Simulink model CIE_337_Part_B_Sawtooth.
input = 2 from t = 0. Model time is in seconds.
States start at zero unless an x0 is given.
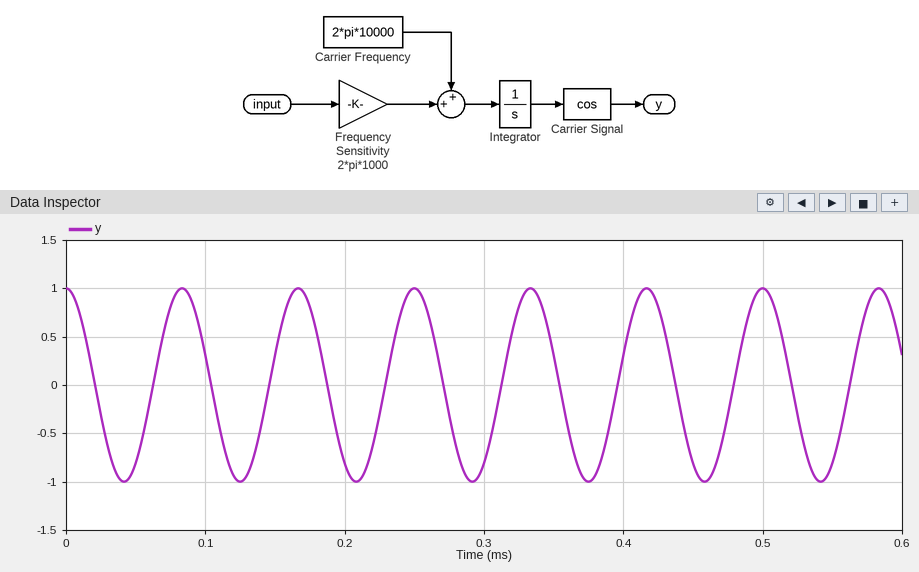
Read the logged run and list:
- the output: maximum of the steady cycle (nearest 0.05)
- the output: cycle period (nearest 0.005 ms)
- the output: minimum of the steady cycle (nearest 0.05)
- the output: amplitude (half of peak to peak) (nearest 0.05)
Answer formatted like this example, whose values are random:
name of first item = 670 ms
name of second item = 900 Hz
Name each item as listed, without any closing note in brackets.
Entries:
the output: maximum of the steady cycle = 1.00
the output: cycle period = 0.085 ms
the output: minimum of the steady cycle = -1.00
the output: amplitude (half of peak to peak) = 1.00
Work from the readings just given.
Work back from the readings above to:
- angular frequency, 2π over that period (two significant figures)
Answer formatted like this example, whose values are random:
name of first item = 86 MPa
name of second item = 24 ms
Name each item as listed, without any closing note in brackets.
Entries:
angular frequency, 2π over that period = 74 rad/ms
